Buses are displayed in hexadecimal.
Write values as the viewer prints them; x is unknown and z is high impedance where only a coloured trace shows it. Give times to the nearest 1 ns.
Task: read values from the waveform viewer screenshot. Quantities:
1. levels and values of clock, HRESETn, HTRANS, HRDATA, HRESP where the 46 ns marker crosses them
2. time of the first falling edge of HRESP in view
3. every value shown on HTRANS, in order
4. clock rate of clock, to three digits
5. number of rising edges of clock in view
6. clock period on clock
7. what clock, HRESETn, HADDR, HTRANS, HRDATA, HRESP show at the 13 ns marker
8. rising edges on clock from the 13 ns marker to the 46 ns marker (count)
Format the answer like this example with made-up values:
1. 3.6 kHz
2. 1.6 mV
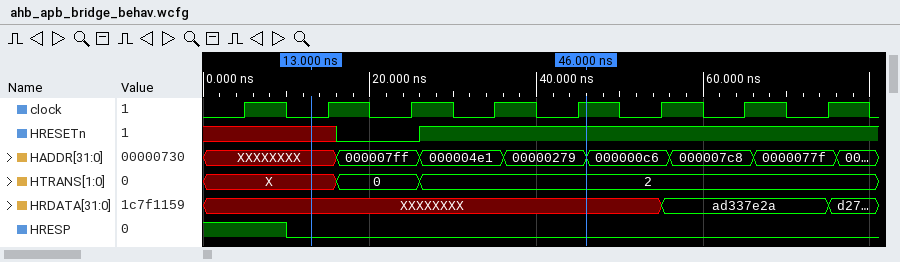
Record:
1. clock=1, HRESETn=1, HTRANS=2, HRDATA=XXXXXXXX, HRESP=0
2. 10 ns
3. X, 0, 2
4. 100 MHz
5. 8
6. 10 ns
7. clock=0, HRESETn=x, HADDR=XXXXXXXX, HTRANS=X, HRDATA=XXXXXXXX, HRESP=0
8. 4
